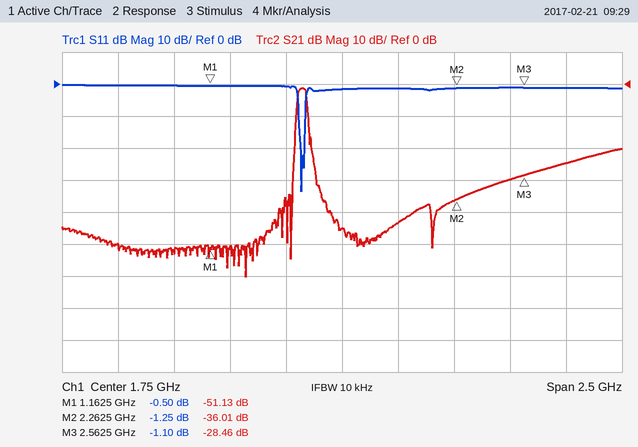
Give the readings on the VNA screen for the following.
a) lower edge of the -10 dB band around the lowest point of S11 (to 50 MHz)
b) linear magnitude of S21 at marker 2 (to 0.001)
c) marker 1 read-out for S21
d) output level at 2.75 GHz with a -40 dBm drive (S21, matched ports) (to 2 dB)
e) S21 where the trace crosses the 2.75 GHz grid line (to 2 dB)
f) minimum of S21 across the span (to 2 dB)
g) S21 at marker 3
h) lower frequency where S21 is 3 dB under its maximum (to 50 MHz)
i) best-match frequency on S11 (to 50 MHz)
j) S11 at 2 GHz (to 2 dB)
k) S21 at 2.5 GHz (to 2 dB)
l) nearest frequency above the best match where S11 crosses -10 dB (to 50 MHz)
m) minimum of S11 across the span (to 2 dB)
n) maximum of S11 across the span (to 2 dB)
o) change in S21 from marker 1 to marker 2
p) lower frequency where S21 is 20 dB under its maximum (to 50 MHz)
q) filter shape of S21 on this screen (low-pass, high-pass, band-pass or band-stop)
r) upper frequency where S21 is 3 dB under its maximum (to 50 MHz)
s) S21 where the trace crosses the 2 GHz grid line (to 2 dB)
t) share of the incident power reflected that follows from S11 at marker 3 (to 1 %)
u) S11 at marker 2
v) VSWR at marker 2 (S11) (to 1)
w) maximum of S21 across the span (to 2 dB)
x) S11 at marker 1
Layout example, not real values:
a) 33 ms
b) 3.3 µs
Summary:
a) 1.55 GHz
b) 0.016
c) -51.13 dB
d) -64 dBm
e) -24 dB
f) -60 dB
g) -28.46 dB
h) 1.55 GHz
i) 1.55 GHz
j) -2 dB
k) -30 dB
l) 1.60 GHz
m) -34 dB
n) 0 dB
o) 15.12 dB
p) 1.55 GHz
q) band-pass
r) 1.60 GHz
s) -44 dB
t) 78 %
u) -1.25 dB
v) 14
w) -2 dB
x) -0.50 dB
